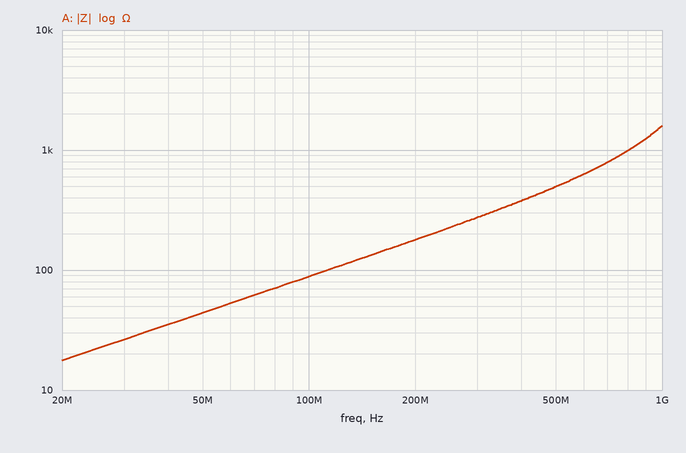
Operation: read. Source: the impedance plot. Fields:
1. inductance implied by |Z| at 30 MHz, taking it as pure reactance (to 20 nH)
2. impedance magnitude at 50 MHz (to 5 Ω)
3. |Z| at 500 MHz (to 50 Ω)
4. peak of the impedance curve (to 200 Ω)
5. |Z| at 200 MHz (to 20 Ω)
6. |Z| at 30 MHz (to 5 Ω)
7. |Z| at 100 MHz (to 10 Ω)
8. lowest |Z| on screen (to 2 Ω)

140 nH
45 Ω
500 Ω
1.6 kΩ
180 Ω
25 Ω
90 Ω
18 Ω
